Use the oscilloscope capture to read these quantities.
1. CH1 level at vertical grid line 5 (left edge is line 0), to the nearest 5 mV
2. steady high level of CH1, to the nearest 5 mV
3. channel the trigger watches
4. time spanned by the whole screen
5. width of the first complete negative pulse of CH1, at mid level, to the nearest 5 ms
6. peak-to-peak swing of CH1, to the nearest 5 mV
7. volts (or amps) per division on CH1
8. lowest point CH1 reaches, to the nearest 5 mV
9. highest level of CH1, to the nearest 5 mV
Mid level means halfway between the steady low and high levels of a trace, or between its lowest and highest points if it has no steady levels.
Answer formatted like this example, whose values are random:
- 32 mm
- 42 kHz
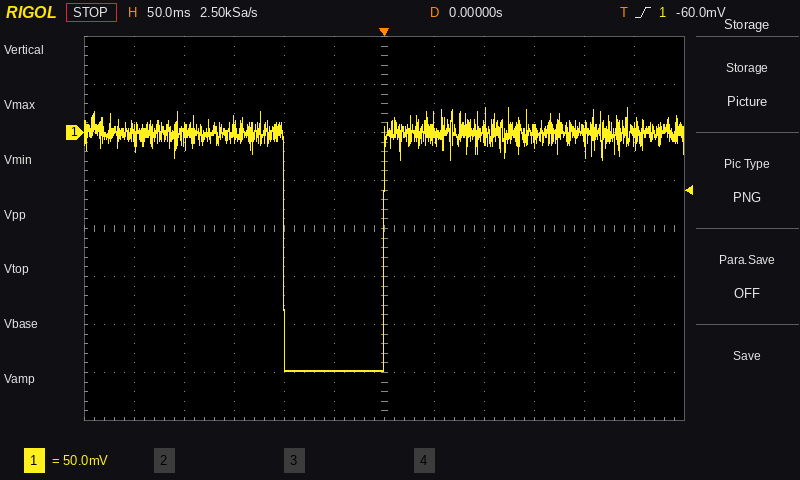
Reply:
- -250 mV
- 0 mV
- CH1
- 600 ms
- 100 ms
- 275 mV
- 50 mV
- -250 mV
- 25 mV
